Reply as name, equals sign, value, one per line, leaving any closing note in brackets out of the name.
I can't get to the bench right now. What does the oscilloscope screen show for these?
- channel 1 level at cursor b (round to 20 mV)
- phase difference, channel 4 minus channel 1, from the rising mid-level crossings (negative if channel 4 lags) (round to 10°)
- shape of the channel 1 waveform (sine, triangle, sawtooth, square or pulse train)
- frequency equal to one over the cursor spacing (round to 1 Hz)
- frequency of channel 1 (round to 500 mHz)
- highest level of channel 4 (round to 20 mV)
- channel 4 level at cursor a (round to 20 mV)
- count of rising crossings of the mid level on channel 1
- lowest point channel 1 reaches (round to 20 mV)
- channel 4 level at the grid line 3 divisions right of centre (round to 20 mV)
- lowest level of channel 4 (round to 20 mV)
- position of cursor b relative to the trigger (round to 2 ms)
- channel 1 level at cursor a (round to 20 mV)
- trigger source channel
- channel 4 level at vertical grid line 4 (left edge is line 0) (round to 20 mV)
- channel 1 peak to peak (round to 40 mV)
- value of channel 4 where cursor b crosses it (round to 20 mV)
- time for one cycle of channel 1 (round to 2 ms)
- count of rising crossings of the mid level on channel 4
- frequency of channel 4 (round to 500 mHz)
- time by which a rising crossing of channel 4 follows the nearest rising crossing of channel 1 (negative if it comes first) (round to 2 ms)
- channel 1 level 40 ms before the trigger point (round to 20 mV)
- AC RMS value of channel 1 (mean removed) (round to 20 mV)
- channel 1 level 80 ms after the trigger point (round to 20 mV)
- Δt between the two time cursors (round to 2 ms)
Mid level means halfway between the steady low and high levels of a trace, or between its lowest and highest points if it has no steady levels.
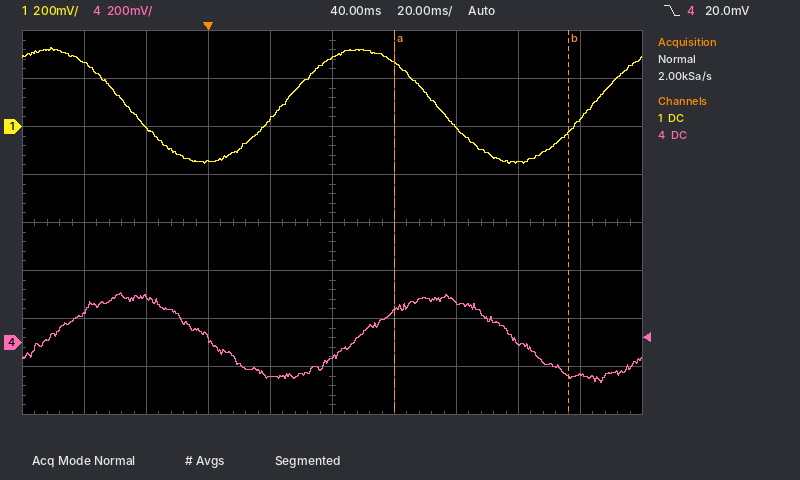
channel 1 level at cursor b = -20 mV
phase difference, channel 4 minus channel 1, from the rising mid-level crossings (negative if channel 4 lags) = -90°
shape of the channel 1 waveform = sine
frequency equal to one over the cursor spacing = 18 Hz
frequency of channel 1 = 10.0 Hz
highest level of channel 4 = 200 mV
channel 4 level at cursor a = 140 mV
count of rising crossings of the mid level on channel 1 = 2
lowest point channel 1 reaches = -160 mV
channel 4 level at the grid line 3 divisions right of centre = 0 mV
lowest level of channel 4 = -160 mV
position of cursor b relative to the trigger = +116 ms
channel 1 level at cursor a = 260 mV
trigger source channel = channel 4
channel 4 level at vertical grid line 4 (left edge is line 0) = -140 mV
channel 1 peak to peak = 480 mV
value of channel 4 where cursor b crosses it = -140 mV
time for one cycle of channel 1 = 100 ms
count of rising crossings of the mid level on channel 4 = 2
frequency of channel 4 = 10.0 Hz
time by which a rising crossing of channel 4 follows the nearest rising crossing of channel 1 (negative if it comes first) = +24 ms
channel 1 level 40 ms before the trigger point = 260 mV
AC RMS value of channel 1 (mean removed) = 160 mV
channel 1 level 80 ms after the trigger point = 0 mV
Δt between the two time cursors = 56 ms
